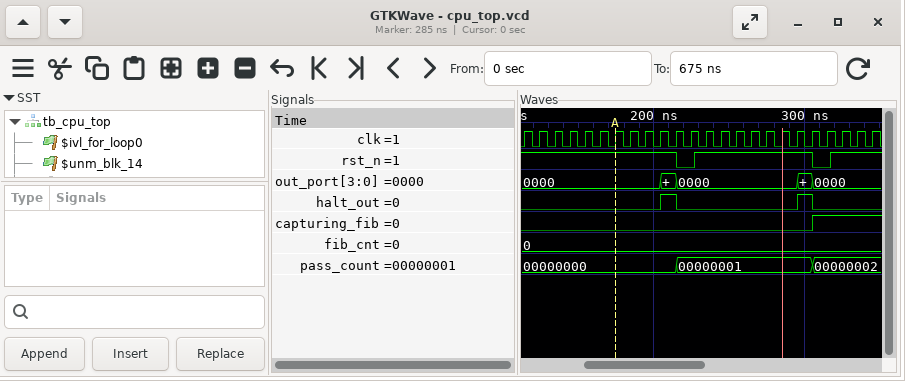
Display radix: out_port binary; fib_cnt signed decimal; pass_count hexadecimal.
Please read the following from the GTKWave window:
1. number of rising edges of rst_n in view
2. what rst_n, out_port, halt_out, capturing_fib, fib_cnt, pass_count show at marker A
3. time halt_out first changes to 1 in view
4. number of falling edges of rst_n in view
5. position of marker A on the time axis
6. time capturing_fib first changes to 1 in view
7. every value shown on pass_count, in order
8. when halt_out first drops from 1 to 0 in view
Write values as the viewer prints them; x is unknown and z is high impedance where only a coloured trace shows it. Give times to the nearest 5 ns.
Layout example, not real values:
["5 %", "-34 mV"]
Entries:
["2", "rst_n=1, out_port=0000, halt_out=0, capturing_fib=0, fib_cnt=0, pass_count=00000000", "205 ns", "2", "175 ns", "305 ns", "00000000, 00000001, 00000002", "215 ns"]
